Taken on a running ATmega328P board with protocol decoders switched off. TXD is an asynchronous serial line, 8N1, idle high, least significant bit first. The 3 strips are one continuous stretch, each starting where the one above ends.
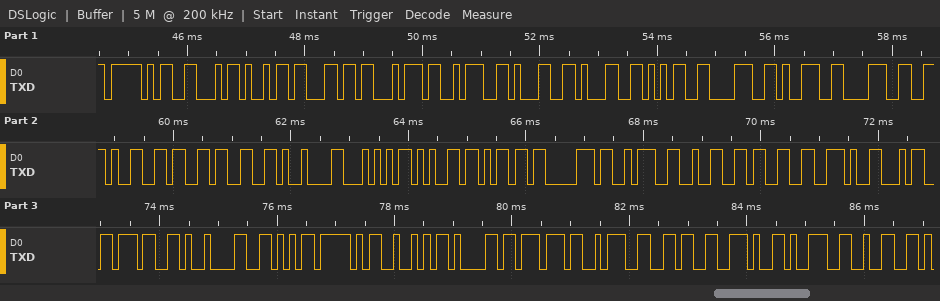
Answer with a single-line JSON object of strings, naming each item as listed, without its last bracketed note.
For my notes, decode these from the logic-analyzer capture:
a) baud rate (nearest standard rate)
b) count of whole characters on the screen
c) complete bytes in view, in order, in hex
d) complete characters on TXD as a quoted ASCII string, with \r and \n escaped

{"baud rate": "9600 baud", "count of whole characters on the screen": "37", "complete bytes in view, in order, in hex": "5F 46 69 6C 74 3A 31 31 35 38 39 38 2E 36 33 09 54 65 6D 70 3A 32 33 2E 34 37 09 56 5F 52 61 77 3A 36 2E 39 32", "complete characters on TXD as a quoted ASCII string, with \\r and \\n escaped": "\"_Filt:115898.63\\tTemp:23.47\\tV_Raw:6.92\""}
